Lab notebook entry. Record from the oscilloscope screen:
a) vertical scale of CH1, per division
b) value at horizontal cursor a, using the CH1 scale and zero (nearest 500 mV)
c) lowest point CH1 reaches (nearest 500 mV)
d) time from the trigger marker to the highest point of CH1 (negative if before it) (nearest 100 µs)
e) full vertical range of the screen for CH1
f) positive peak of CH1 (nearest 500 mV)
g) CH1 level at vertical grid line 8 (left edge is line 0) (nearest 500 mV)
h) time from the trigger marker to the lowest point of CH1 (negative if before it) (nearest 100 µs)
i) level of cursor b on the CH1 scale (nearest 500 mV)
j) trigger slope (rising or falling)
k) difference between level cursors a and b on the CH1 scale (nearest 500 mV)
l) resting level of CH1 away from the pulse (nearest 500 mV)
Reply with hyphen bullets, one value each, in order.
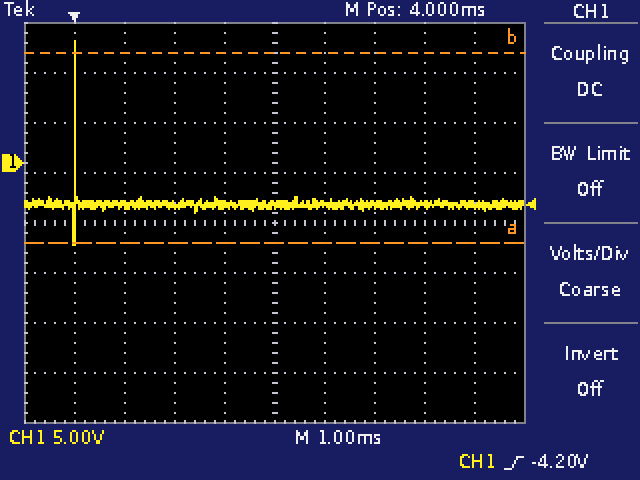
- 5 V
- -8.0 V
- -8.0 V
- 0.0 ms
- 40 V
- 12.0 V
- -4.0 V
- 0.0 ms
- 11.0 V
- rising
- 19.0 V
- -4.0 V
